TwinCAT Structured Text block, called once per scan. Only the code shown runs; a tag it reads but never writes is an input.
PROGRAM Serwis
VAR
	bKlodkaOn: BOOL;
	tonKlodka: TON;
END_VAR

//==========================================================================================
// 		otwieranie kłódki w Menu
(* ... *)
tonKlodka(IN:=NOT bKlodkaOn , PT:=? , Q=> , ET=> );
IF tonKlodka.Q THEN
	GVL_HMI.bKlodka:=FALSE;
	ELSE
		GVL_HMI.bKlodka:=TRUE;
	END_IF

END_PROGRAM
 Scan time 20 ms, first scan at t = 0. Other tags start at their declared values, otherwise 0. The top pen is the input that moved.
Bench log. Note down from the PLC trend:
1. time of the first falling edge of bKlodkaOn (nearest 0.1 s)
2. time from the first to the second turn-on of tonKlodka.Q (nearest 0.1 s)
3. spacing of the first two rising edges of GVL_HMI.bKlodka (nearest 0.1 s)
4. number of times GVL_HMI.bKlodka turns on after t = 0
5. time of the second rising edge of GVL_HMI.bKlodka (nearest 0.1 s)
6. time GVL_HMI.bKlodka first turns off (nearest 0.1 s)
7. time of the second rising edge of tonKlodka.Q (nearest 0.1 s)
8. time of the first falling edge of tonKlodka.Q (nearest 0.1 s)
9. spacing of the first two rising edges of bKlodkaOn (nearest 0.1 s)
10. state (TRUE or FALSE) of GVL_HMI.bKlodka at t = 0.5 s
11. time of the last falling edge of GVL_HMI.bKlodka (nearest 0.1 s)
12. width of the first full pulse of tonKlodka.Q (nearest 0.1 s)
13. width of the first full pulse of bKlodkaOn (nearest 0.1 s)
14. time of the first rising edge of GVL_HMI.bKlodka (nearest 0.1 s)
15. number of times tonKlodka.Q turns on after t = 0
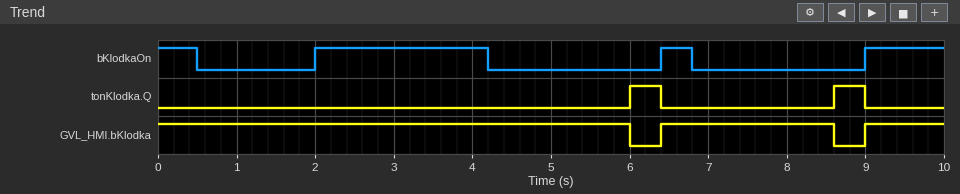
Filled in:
0.5 s
2.6 s
2.6 s
2
9.0 s
6.0 s
8.6 s
6.4 s
4.4 s
TRUE
8.6 s
0.4 s
2.2 s
6.4 s
2
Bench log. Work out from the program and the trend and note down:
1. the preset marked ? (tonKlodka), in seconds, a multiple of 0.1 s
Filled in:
1.8 s
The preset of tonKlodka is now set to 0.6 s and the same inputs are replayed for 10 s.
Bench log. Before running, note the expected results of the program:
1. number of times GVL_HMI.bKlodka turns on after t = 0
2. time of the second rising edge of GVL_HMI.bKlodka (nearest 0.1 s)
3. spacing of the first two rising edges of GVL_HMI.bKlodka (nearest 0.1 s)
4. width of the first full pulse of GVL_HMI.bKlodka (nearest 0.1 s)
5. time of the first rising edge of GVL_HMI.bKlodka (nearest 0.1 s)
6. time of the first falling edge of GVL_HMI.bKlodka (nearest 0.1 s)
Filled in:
3
6.4 s
4.4 s
2.8 s
2.0 s
1.1 s
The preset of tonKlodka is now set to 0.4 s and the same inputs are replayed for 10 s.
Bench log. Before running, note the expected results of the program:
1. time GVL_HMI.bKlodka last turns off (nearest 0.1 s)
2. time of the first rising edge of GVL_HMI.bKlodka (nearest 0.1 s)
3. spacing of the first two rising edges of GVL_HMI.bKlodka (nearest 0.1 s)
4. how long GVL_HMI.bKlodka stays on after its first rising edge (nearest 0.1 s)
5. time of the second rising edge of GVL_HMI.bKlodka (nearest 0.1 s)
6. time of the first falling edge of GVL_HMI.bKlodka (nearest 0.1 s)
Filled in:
7.2 s
2.0 s
4.4 s
2.6 s
6.4 s
0.9 s
